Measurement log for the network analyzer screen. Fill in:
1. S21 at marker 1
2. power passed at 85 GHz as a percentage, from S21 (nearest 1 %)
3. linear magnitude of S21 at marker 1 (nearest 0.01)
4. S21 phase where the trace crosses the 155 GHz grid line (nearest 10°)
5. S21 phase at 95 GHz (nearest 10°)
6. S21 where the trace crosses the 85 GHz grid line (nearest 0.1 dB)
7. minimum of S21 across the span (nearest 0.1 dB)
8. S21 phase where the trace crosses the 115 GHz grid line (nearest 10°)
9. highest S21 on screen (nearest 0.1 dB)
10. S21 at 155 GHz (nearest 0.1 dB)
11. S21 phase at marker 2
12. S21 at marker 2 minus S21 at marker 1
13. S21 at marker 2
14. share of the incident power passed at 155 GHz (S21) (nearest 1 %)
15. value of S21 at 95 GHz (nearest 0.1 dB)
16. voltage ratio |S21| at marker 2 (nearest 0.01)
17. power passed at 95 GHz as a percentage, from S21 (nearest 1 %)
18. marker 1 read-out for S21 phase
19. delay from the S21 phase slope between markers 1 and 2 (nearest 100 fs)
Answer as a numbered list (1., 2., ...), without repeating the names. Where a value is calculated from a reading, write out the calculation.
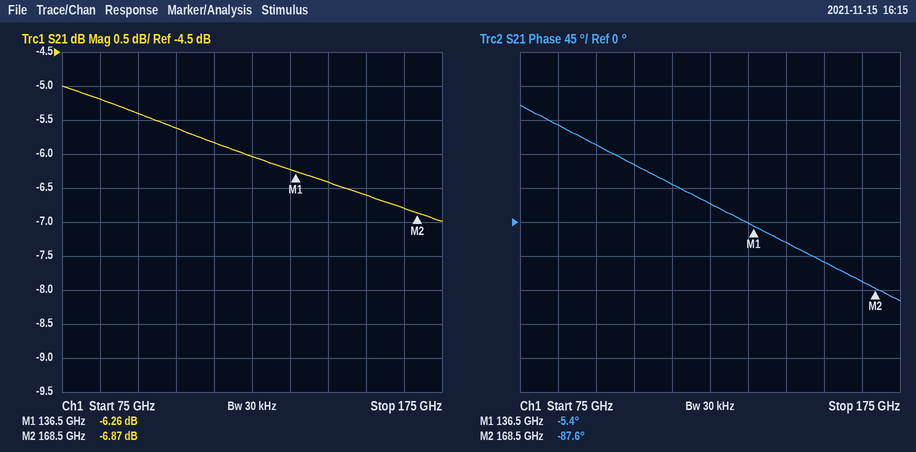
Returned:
1. -6.26 dB
2. 10^(-5.2/10) ≈ 30 %
3. 10^(-6.26/20) ≈ 0.49
4. -50°
5. 100°
6. -5.2 dB
7. -7.0 dB
8. 50°
9. -5.0 dB
10. -6.6 dB
11. -87.6°
12. -6.87 − (-6.26) = -0.61 dB
13. -6.87 dB
14. 10^(-6.6/10) ≈ 22 %
15. -5.4 dB
16. 10^(-6.87/20) ≈ 0.45
17. 10^(-5.4/10) ≈ 29 %
18. -5.4°
19. −(-87.6° − (-5.4°))/(360° × 32 GHz) ≈ 7.1 ps
